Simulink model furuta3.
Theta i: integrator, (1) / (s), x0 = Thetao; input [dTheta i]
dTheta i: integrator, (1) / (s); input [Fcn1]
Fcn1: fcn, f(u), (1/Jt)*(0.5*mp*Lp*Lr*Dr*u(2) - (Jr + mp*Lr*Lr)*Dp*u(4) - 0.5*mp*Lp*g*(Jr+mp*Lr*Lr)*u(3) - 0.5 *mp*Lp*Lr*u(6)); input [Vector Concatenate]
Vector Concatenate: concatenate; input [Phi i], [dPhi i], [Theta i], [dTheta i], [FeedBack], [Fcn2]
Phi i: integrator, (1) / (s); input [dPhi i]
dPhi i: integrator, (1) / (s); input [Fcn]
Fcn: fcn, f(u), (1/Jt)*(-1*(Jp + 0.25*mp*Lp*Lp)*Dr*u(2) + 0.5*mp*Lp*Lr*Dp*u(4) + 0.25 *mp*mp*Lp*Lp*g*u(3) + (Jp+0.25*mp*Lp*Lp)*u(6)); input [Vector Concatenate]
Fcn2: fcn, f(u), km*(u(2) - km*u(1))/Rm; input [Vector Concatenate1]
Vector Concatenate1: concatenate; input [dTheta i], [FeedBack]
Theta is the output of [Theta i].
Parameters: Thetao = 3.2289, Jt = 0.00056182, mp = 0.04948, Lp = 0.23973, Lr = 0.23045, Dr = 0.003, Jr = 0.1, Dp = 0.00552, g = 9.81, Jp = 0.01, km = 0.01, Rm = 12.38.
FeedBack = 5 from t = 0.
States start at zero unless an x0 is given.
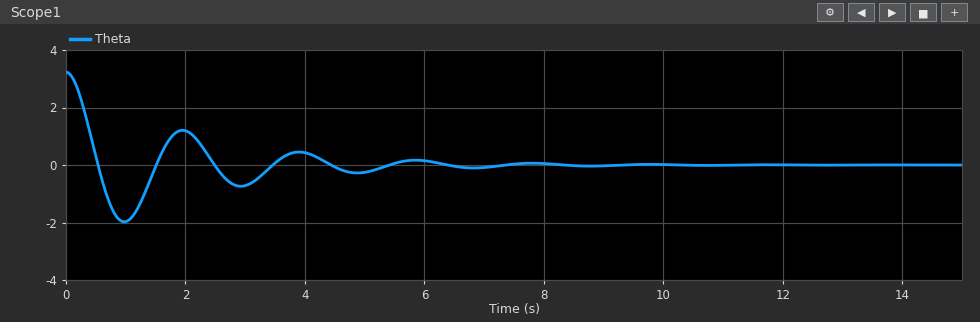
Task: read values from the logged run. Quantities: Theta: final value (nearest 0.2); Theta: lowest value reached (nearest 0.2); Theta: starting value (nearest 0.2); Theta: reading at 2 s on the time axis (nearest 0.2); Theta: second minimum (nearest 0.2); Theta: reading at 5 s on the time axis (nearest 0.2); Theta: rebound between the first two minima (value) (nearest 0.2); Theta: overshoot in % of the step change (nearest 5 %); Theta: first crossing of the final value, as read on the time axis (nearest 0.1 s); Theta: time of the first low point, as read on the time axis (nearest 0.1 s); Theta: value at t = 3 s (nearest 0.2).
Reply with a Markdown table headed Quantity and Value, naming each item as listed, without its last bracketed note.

| Quantity | Value |
|---|---|
| Theta: final value | 0.0 |
| Theta: lowest value reached | -2.0 |
| Theta: starting value | 3.2 |
| Theta: reading at 2 s on the time axis | 1.2 |
| Theta: second minimum | -0.8 |
| Theta: reading at 5 s on the time axis | -0.2 |
| Theta: rebound between the first two minima (value) | 1.2 |
| Theta: overshoot in % of the step change | 60 % |
| Theta: first crossing of the final value, as read on the time axis | 0.5 s |
| Theta: time of the first low point, as read on the time axis | 1.0 s |
| Theta: value at t = 3 s | -0.8 |
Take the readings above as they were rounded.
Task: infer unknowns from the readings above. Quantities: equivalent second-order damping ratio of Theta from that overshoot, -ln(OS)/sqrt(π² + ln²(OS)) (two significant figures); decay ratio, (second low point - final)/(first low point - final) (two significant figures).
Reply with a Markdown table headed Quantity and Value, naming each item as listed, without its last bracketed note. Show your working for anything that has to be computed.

| Quantity | Value |
|---|---|
| equivalent second-order damping ratio of Theta from that overshoot, -ln(OS)/sqrt(π² + ln²(OS)) | ln(0.6) = -0.511; 0.511 / sqrt(9.870 + 0.261) = 0.16 |
| decay ratio, (second low point - final)/(first low point - final) | (-0.8 - 0) / (-2 - 0) = 0.40 |
